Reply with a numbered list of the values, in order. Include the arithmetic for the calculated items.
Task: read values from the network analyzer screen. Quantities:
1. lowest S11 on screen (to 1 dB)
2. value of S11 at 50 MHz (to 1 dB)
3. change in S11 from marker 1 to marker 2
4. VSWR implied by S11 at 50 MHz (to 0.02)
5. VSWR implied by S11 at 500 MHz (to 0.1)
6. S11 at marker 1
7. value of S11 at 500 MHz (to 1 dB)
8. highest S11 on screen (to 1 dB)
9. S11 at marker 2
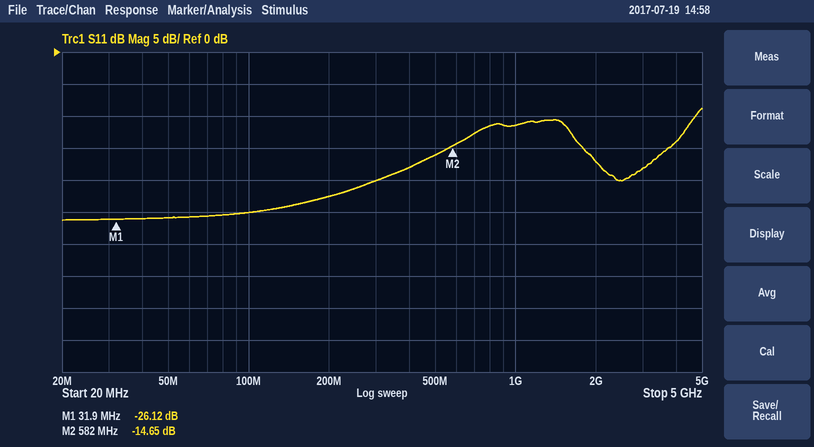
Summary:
1. -26 dB
2. -26 dB
3. -14.65 − (-26.12) = 11.47 dB
4. |Γ| = 10^(-26/20) = 0.0501; VSWR = (1 + 0.0501)/(1 − 0.0501) ≈ 1.11, so 1.10 to the nearest 0.02
5. |Γ| = 10^(-16/20) = 0.1585; VSWR = (1 + 0.1585)/(1 − 0.1585) ≈ 1.4
6. -26.12 dB
7. -16 dB
8. -9 dB
9. -14.65 dB
